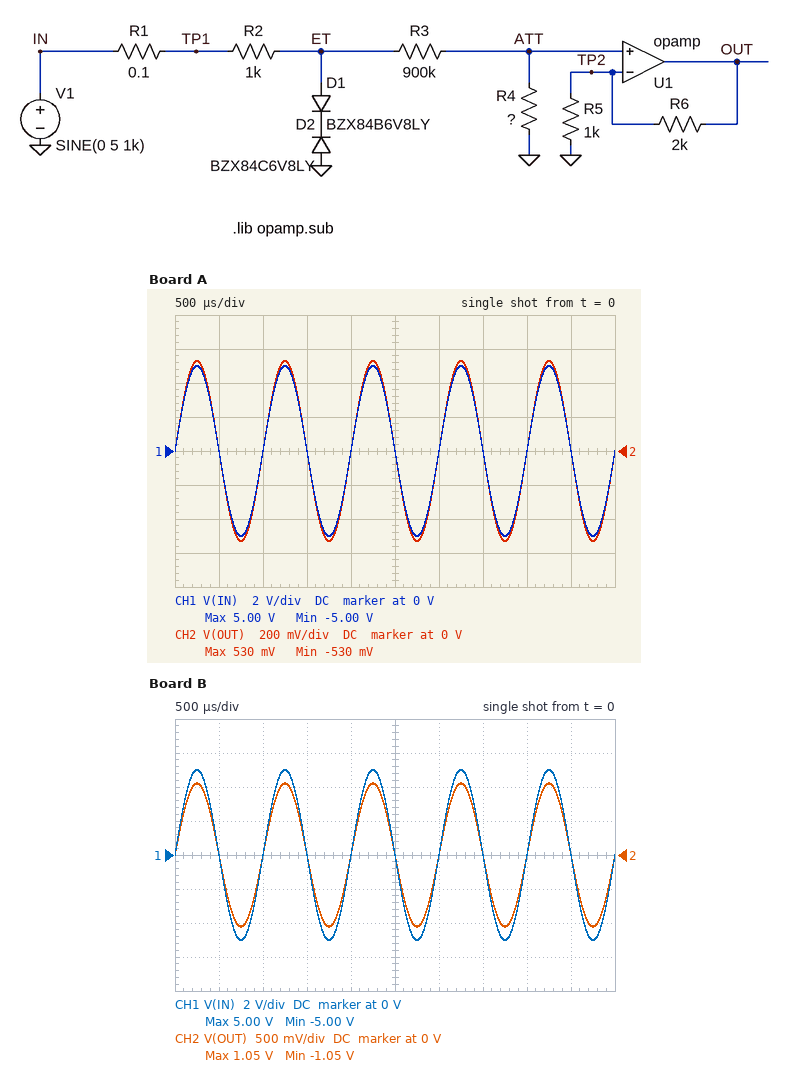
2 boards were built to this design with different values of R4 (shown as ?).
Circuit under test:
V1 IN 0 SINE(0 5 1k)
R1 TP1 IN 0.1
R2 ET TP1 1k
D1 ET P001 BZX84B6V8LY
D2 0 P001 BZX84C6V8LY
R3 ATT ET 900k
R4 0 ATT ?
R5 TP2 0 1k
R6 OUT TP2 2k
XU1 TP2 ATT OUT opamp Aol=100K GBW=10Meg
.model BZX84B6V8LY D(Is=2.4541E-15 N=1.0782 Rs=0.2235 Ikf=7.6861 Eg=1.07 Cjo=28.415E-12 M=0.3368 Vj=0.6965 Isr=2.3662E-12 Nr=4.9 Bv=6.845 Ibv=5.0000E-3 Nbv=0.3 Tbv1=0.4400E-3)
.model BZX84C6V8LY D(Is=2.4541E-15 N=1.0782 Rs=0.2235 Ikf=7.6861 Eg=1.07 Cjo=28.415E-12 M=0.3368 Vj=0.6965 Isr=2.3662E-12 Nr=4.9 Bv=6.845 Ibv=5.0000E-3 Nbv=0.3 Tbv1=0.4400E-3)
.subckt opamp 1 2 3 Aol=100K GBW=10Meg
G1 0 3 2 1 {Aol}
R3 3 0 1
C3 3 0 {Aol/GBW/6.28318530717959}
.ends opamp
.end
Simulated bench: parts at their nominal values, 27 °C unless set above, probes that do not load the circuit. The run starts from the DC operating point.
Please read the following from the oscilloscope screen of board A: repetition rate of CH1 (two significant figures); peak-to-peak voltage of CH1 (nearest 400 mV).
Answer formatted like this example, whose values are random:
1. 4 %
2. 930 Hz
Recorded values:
1. 1.0 kHz
2. 10.0 V
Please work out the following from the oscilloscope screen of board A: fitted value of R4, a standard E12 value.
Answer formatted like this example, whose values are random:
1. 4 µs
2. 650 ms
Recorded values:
1. 33 kΩ
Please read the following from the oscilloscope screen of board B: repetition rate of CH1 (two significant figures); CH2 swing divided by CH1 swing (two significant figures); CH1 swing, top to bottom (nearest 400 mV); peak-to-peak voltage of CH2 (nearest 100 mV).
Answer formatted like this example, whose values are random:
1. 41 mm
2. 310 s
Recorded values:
1. 1.0 kHz
2. 0.21
3. 10.0 V
4. 2.1 V
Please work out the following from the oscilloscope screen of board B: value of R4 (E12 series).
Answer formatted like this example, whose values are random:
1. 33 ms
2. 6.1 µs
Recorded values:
1. 68 kΩ
